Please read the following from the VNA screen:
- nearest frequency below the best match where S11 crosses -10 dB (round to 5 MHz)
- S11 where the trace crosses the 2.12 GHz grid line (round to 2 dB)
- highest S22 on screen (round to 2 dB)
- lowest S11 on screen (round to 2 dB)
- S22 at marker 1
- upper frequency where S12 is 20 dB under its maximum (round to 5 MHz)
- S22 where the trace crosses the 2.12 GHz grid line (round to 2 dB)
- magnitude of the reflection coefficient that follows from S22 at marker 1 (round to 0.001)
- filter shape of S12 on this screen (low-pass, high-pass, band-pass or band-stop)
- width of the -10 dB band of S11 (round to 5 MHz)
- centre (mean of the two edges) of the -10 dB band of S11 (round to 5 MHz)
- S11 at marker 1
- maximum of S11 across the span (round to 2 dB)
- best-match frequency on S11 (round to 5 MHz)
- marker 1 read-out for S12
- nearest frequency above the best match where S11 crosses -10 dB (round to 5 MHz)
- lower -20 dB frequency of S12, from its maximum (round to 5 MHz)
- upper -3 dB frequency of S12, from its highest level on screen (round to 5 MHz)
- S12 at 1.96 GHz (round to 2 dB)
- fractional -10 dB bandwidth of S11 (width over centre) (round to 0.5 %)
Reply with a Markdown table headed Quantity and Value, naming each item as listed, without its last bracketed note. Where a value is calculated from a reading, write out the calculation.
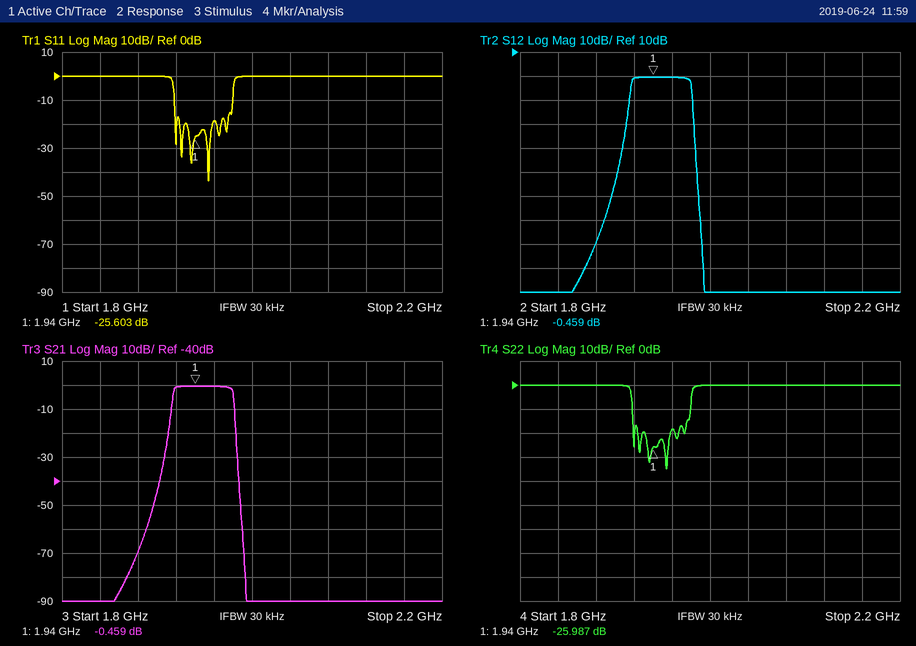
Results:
| Quantity | Value |
|---|---|
| nearest frequency below the best match where S11 crosses -10 dB | 1.920 GHz |
| S11 where the trace crosses the 2.12 GHz grid line | 0 dB |
| highest S22 on screen | 0 dB |
| lowest S11 on screen | -44 dB |
| S22 at marker 1 | -25.987 dB |
| upper frequency where S12 is 20 dB under its maximum | 1.985 GHz |
| S22 where the trace crosses the 2.12 GHz grid line | 0 dB |
| magnitude of the reflection coefficient that follows from S22 at marker 1 | 10^(-25.987/20) ≈ 0.050 |
| filter shape of S12 on this screen | band-pass |
| width of the -10 dB band of S11 | 1.980 GHz − 1.920 GHz = 60 MHz |
| centre (mean of the two edges) of the -10 dB band of S11 | 1.950 GHz |
| S11 at marker 1 | -25.603 dB |
| maximum of S11 across the span | 0 dB |
| best-match frequency on S11 | 1.955 GHz |
| marker 1 read-out for S12 | -0.459 dB |
| nearest frequency above the best match where S11 crosses -10 dB | 1.980 GHz |
| lower -20 dB frequency of S12, from its maximum | 1.910 GHz |
| upper -3 dB frequency of S12, from its highest level on screen | 1.980 GHz |
| S12 at 1.96 GHz | 0 dB |
| fractional -10 dB bandwidth of S11 (width over centre) | 60 MHz / 1.95 GHz ≈ 3.08 %, so 3.0 % to the nearest 0.5 % |
